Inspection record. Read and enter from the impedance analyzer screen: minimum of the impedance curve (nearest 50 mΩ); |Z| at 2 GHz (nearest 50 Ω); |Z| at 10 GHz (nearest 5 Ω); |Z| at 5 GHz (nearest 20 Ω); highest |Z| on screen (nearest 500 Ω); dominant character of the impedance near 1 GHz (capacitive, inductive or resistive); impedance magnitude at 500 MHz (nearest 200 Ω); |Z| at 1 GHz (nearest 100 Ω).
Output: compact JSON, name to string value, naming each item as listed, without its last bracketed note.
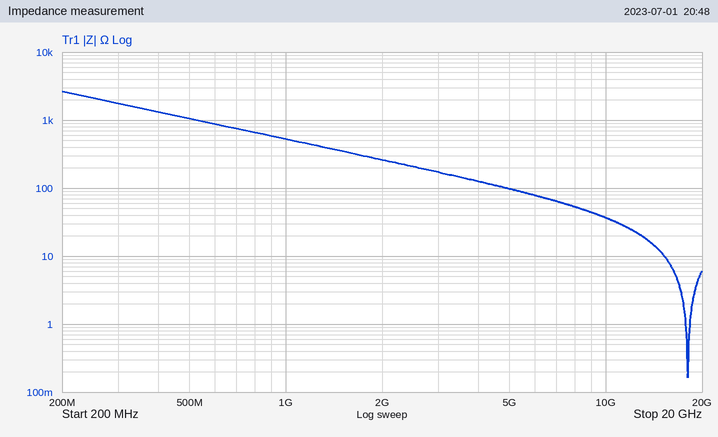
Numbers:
{"minimum of the impedance curve": "150 mΩ", "|Z| at 2 GHz": "250 Ω", "|Z| at 10 GHz": "35 Ω", "|Z| at 5 GHz": "100 Ω", "highest |Z| on screen": "2.5 kΩ", "dominant character of the impedance near 1 GHz": "capacitive", "impedance magnitude at 500 MHz": "1.0 kΩ", "|Z| at 1 GHz": "500 Ω"}
